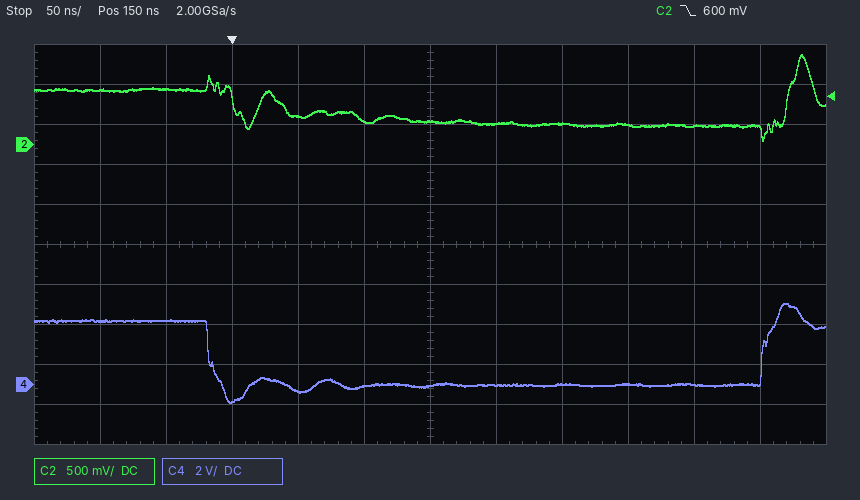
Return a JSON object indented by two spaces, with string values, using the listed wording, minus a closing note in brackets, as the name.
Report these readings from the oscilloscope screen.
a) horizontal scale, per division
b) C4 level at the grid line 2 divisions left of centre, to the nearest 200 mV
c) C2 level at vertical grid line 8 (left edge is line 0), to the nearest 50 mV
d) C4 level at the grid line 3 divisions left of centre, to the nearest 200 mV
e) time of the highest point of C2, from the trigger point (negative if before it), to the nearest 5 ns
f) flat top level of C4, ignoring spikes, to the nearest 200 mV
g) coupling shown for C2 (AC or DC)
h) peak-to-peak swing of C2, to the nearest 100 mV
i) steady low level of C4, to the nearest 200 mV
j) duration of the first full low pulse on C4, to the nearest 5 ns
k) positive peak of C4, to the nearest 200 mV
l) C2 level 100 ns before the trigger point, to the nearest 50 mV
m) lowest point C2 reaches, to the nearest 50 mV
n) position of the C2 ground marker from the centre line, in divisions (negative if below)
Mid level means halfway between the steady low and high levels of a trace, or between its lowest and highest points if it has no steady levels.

{
  "horizontal scale, per division": "50 ns",
  "C4 level at the grid line 2 divisions left of centre, to the nearest 200 mV": "-400 mV",
  "C2 level at vertical grid line 8 (left edge is line 0), to the nearest 50 mV": "250 mV",
  "C4 level at the grid line 3 divisions left of centre, to the nearest 200 mV": "-800 mV",
  "time of the highest point of C2, from the trigger point (negative if before it), to the nearest 5 ns": "+430 ns",
  "flat top level of C4, ignoring spikes, to the nearest 200 mV": "3.2 V",
  "coupling shown for C2": "DC",
  "peak-to-peak swing of C2, to the nearest 100 mV": "1.10 V",
  "steady low level of C4, to the nearest 200 mV": "0.0 V",
  "duration of the first full low pulse on C4, to the nearest 5 ns": "420 ns",
  "positive peak of C4, to the nearest 200 mV": "4.0 V",
  "C2 level 100 ns before the trigger point, to the nearest 50 mV": "700 mV",
  "lowest point C2 reaches, to the nearest 50 mV": "50 mV",
  "position of the C2 ground marker from the centre line, in divisions": "+2.5 div"
}
